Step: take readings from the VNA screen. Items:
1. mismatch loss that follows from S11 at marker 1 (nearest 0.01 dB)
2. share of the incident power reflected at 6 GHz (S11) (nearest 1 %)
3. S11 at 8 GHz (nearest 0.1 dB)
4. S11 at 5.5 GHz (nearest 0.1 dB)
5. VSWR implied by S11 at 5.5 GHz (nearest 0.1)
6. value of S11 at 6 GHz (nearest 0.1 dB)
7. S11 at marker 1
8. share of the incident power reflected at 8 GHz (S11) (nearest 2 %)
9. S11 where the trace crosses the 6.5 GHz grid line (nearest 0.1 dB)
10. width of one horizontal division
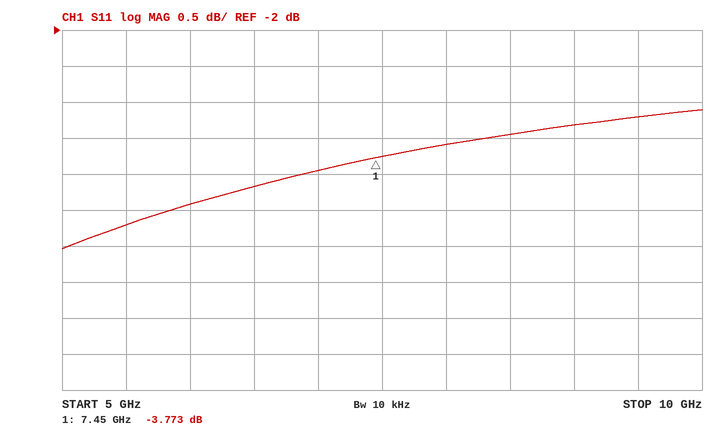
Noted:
2.36 dB
36 %
-3.6 dB
-4.7 dB
3.8
-4.4 dB
-3.773 dB
44 %
-4.2 dB
500 MHz
